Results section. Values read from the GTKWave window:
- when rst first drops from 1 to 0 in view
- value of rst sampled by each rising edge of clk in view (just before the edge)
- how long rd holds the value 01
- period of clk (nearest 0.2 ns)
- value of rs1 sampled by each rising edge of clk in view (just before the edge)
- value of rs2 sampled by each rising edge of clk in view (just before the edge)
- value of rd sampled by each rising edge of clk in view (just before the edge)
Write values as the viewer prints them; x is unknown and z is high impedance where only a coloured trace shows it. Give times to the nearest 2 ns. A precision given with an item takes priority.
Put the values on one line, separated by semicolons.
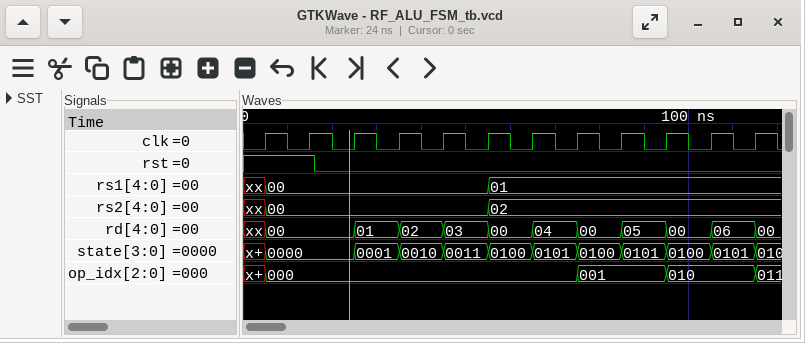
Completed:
16 ns; 1 1 0 0 0 0 0 0 0 0 0 0; 10 ns; 10 ns; xx, 00, 00, 00, 00, 00, 01, 01, 01, 01, 01, 01; xx, 00, 00, 00, 00, 00, 02, 02, 02, 02, 02, 02; xx, 00, 00, 01, 02, 03, 00, 04, 00, 05, 00, 06
